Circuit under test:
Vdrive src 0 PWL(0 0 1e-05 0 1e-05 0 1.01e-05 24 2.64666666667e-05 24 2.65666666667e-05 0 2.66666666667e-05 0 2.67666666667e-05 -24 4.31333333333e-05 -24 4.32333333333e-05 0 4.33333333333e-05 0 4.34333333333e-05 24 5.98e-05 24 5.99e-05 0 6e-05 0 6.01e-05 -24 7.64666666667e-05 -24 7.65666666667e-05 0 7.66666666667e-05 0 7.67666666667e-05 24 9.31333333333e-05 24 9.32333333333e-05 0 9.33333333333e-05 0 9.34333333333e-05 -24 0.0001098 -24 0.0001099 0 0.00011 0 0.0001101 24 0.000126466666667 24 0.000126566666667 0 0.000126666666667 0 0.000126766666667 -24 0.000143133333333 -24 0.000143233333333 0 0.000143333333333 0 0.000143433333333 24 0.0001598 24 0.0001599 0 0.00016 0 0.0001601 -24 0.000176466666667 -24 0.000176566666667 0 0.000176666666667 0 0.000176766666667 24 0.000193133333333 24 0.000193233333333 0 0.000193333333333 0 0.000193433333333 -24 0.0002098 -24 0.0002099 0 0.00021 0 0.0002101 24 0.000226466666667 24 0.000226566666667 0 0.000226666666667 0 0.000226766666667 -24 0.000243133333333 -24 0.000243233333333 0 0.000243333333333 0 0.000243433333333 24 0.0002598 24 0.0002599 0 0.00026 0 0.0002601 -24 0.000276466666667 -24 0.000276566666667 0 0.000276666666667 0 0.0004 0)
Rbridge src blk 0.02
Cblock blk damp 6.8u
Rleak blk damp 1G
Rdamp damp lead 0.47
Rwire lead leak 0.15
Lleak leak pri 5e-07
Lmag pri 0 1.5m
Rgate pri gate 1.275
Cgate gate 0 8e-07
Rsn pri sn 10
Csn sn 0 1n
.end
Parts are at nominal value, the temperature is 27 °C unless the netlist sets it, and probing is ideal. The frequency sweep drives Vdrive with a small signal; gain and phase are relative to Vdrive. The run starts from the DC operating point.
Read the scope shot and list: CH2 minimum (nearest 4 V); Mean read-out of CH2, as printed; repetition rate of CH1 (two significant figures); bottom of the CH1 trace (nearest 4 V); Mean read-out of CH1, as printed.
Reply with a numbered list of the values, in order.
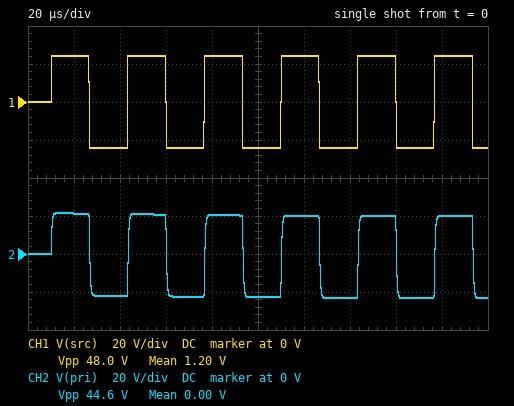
1. -24 V
2. 0.00 V
3. 30 kHz
4. -24 V
5. 1.20 V
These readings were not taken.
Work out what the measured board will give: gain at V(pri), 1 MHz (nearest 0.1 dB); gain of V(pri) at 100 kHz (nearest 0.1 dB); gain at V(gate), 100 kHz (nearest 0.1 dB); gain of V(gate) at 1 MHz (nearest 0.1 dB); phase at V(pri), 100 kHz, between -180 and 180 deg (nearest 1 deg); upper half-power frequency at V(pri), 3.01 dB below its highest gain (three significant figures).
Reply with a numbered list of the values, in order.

1. -8.6 dB
2. -1.2 dB
3. -2.7 dB
4. -24.9 dB
5. -12 deg
6. 1.52 kHz
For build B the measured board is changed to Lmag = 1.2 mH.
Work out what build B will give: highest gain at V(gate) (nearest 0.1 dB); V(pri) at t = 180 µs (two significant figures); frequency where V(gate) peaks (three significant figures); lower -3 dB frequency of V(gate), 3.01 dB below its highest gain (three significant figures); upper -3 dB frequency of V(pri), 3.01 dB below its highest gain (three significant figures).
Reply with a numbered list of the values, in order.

1. 26.6 dB
2. 20 V
3. 1.67 kHz
4. 1.63 kHz
5. 1.70 kHz
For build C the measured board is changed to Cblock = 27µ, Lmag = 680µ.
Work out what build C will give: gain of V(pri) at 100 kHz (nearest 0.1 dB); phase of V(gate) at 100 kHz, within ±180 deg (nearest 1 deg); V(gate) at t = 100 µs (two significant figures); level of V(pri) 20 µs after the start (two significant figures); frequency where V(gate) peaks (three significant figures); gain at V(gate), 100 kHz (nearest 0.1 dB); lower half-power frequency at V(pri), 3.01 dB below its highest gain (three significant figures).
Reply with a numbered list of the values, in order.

1. -0.8 dB
2. -48 deg
3. -24 V
4. 23 V
5. 1.16 kHz
6. -2.3 dB
7. 1.10 kHz
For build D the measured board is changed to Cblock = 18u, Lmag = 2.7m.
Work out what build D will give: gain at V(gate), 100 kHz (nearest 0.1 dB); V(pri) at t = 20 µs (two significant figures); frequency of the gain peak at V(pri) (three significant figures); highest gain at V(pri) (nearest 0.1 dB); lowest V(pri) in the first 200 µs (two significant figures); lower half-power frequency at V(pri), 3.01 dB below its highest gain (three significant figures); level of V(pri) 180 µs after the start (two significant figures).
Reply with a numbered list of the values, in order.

1. -2.3 dB
2. 23 V
3. 707 Hz
4. 25.8 dB
5. -24 V
6. 690 Hz
7. 22 V
